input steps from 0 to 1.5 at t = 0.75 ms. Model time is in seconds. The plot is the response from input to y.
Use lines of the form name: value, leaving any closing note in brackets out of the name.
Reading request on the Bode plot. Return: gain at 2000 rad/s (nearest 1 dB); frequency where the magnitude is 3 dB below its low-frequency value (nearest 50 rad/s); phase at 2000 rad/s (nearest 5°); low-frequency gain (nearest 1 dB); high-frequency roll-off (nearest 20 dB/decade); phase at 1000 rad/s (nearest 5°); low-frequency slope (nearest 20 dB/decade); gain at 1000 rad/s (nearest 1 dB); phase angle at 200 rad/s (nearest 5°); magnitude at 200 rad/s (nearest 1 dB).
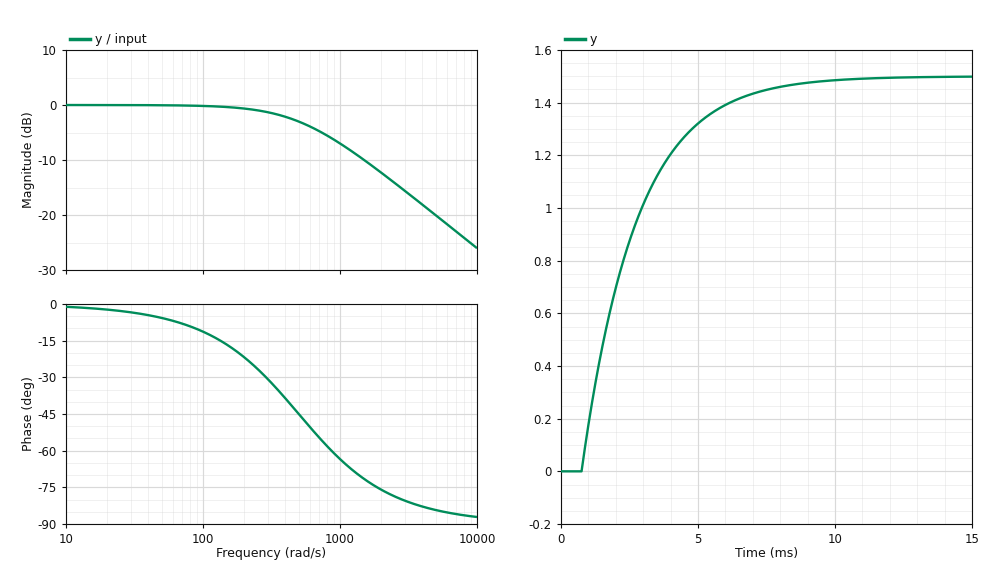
gain at 2000 rad/s: -12 dB
frequency where the magnitude is 3 dB below its low-frequency value: 500 rad/s
phase at 2000 rad/s: -75°
low-frequency gain: 0 dB
high-frequency roll-off: -20 dB/decade
phase at 1000 rad/s: -65°
low-frequency slope: 0 dB/decade
gain at 1000 rad/s: -7 dB
phase angle at 200 rad/s: -20°
magnitude at 200 rad/s: -1 dB
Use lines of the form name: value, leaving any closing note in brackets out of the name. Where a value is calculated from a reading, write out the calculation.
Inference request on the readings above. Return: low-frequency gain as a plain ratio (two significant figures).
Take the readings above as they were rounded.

low-frequency gain as a plain ratio: 10^(0 / 20) = 1.0
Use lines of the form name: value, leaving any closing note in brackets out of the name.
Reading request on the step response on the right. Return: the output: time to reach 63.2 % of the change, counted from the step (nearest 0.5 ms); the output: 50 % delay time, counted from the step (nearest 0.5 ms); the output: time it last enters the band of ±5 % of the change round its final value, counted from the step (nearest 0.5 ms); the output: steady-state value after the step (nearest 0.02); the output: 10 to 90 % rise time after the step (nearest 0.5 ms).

the output: time to reach 63.2 % of the change, counted from the step: 2.0 ms
the output: 50 % delay time, counted from the step: 1.5 ms
the output: time it last enters the band of ±5 % of the change round its final value, counted from the step: 6.0 ms
the output: steady-state value after the step: 1.50
the output: 10 to 90 % rise time after the step: 4.5 ms
